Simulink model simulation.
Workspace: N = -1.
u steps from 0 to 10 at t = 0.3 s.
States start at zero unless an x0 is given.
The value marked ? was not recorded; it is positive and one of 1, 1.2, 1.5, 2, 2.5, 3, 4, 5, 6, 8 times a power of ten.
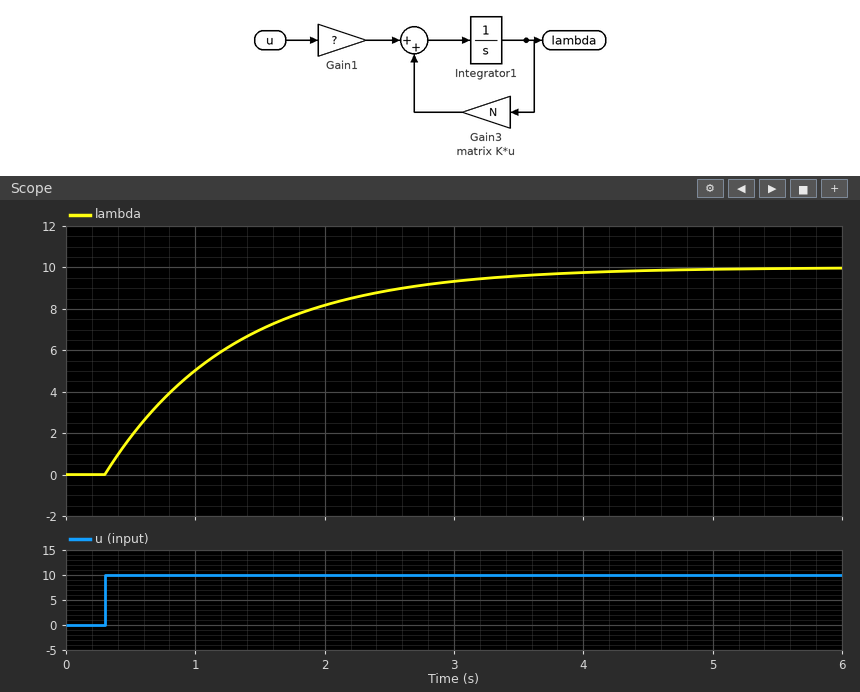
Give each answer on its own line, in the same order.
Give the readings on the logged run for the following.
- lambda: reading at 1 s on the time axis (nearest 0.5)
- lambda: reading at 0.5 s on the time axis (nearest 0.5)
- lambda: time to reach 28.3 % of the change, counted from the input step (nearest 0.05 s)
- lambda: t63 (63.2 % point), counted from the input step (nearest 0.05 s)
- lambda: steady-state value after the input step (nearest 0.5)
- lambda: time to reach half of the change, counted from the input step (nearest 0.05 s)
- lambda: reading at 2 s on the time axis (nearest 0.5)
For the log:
5.0
2.0
0.35 s
1.00 s
10.0
0.70 s
8.0
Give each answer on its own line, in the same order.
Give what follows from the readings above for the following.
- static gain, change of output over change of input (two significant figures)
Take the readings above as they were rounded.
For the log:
1.0
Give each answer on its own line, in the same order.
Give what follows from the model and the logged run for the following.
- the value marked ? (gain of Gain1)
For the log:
1
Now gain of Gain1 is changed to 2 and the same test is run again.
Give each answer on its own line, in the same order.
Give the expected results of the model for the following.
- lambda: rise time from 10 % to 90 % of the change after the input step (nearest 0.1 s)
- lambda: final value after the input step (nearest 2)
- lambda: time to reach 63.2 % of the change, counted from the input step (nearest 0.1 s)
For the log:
2.2 s
20
1.0 s
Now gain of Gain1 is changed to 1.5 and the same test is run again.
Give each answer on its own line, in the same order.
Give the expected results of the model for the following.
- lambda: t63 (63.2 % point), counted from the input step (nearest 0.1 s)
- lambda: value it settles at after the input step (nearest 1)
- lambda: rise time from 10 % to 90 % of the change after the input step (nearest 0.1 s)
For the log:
1.0 s
15
2.2 s
